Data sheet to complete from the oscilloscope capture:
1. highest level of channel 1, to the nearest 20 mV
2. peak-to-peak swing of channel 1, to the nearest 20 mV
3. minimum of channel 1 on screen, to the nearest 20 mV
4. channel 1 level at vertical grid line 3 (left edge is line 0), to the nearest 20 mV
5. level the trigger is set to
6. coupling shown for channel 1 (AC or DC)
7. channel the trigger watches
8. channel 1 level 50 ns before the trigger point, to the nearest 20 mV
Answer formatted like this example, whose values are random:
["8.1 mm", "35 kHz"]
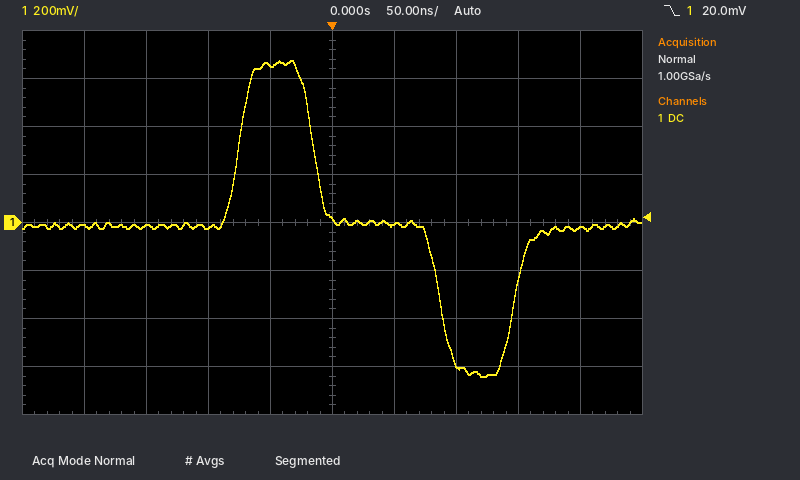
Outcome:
["680 mV", "1.32 V", "-640 mV", "-20 mV", "20.0 mV", "DC", "channel 1", "660 mV"]
